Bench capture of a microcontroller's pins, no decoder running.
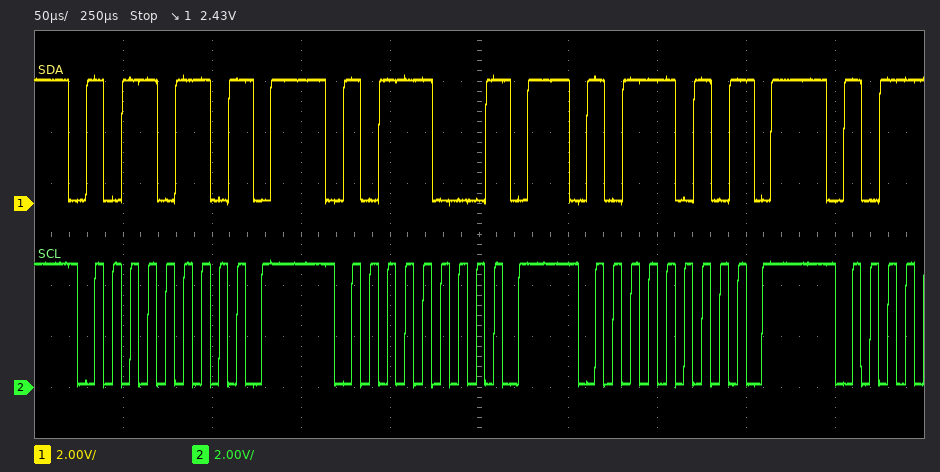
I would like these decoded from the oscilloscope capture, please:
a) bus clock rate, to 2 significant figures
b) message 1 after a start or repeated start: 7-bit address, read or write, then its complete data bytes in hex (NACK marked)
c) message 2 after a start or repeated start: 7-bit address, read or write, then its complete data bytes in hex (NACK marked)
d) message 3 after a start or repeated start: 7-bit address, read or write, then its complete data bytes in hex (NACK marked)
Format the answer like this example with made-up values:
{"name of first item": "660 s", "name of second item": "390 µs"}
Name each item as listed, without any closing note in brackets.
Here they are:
{"bus clock rate, to 2 significant figures": "100 kHz", "message 1 after a start or repeated start: 7-bit address, read or write, then its complete data bytes in hex": "0x5B write NACK", "message 2 after a start or repeated start: 7-bit address, read or write, then its complete data bytes in hex": "0x5C write NACK", "message 3 after a start or repeated start: 7-bit address, read or write, then its complete data bytes in hex": "0x5D write NACK"}
